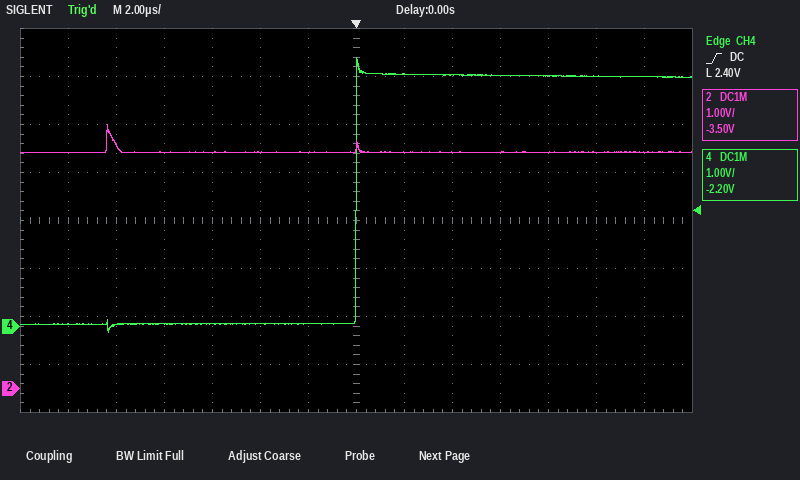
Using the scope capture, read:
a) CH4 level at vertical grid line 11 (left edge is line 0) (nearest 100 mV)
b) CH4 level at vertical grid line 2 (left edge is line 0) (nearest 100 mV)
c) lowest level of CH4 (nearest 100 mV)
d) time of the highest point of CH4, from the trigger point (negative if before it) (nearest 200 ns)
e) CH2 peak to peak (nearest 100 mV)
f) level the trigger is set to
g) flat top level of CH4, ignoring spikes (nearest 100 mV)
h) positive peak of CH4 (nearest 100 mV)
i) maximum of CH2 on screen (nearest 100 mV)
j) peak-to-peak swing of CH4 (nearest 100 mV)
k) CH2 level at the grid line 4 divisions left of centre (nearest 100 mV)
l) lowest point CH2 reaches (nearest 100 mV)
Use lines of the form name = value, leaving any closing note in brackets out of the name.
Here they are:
CH4 level at vertical grid line 11 (left edge is line 0) = 5.2 V
CH4 level at vertical grid line 2 (left edge is line 0) = 0.0 V
lowest level of CH4 = -100 mV
time of the highest point of CH4, from the trigger point (negative if before it) = 0.0 µs
CH2 peak to peak = 600 mV
level the trigger is set to = 2.40 V
flat top level of CH4, ignoring spikes = 5.2 V
positive peak of CH4 = 5.6 V
maximum of CH2 on screen = 5.5 V
peak-to-peak swing of CH4 = 5.7 V
CH2 level at the grid line 4 divisions left of centre = 4.9 V
lowest point CH2 reaches = 4.9 V
